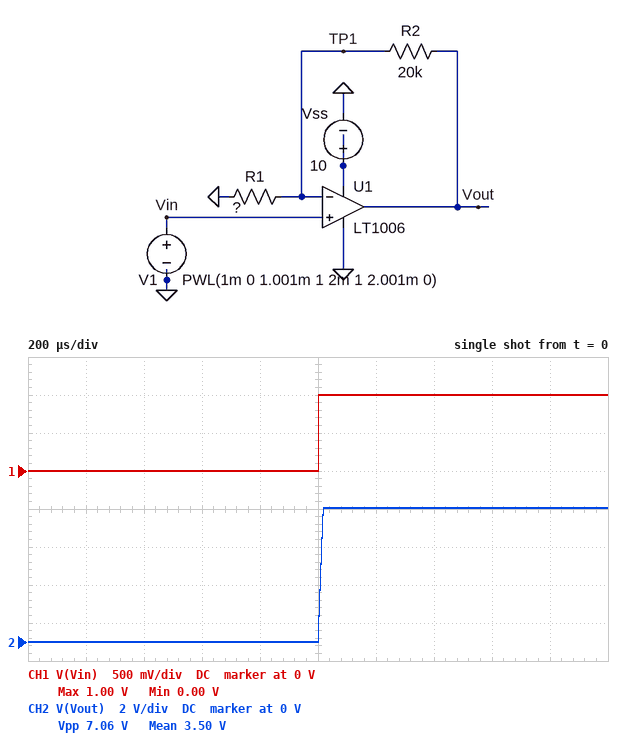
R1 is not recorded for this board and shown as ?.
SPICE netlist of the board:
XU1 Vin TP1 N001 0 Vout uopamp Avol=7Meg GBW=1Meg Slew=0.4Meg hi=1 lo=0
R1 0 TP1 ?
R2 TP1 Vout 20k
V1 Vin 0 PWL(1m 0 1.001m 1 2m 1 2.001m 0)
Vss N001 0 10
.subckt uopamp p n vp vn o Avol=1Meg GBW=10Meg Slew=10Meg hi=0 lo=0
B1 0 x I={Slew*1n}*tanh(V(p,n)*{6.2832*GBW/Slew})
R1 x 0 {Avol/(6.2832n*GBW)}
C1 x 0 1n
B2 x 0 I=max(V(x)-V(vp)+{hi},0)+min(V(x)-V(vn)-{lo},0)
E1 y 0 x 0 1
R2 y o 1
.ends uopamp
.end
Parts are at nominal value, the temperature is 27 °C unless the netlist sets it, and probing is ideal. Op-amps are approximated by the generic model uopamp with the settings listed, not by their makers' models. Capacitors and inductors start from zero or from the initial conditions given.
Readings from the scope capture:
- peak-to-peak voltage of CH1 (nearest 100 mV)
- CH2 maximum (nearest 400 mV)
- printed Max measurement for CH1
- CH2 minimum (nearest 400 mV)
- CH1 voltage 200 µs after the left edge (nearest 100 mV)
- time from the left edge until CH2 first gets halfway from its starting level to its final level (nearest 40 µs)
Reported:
1.0 V
7.2 V
1.00 V
0 V
0 V
1.00 ms
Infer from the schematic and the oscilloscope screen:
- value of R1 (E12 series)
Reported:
3.3 kΩ
